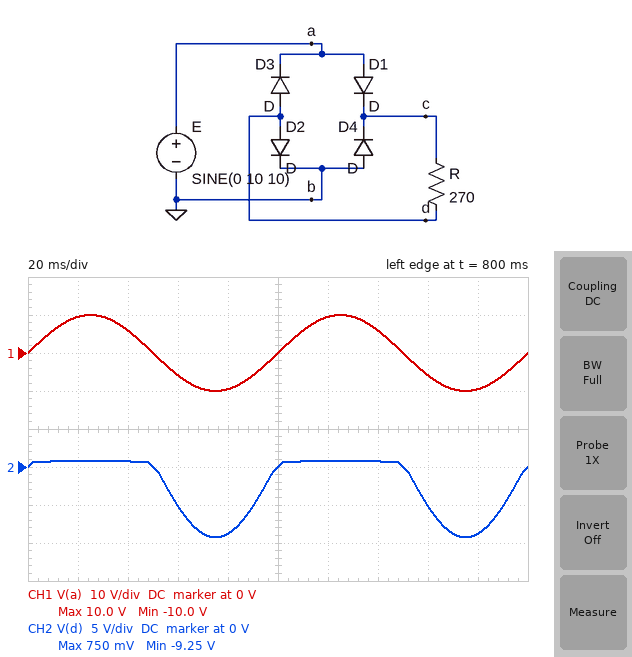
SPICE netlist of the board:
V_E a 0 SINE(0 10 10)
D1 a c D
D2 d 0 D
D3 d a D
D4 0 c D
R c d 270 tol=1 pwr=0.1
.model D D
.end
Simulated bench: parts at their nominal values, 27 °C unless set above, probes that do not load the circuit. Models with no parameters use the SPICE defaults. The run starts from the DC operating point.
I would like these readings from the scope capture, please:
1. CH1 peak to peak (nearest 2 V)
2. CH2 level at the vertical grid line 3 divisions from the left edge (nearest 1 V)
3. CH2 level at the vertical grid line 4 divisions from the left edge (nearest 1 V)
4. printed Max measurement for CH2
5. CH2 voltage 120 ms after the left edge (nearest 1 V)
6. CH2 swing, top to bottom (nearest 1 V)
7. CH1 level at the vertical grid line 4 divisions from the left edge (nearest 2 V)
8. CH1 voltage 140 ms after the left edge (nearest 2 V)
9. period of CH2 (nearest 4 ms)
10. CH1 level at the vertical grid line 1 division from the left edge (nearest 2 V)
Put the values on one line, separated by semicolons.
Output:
20 V; -5 V; -9 V; 750 mV; 1 V; 10 V; -10 V; 6 V; 100 ms; 10 V
